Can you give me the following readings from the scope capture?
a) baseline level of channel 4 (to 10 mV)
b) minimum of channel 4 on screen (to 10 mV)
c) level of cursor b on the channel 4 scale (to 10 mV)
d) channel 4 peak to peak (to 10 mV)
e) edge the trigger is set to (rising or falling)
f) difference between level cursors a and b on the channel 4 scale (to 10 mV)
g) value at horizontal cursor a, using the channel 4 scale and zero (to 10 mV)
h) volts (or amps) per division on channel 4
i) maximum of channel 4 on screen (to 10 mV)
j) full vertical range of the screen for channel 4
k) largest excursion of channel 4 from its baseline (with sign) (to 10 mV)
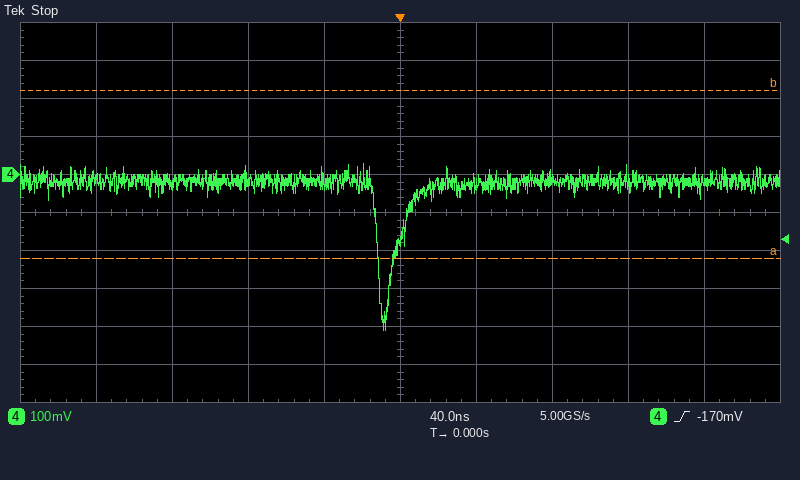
-20 mV
-410 mV
220 mV
440 mV
rising
440 mV
-220 mV
100 mV
30 mV
1 V
-390 mV
